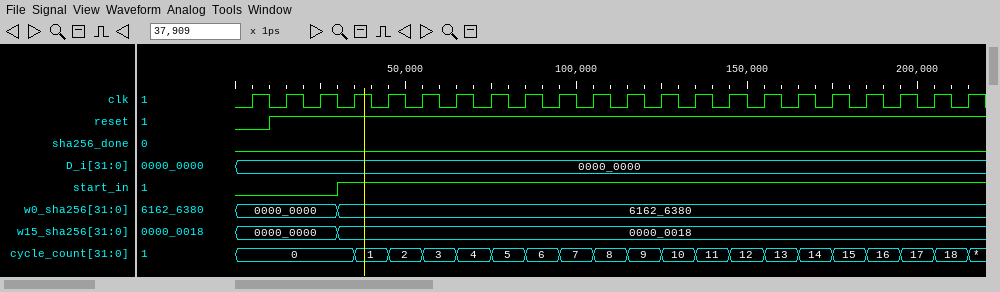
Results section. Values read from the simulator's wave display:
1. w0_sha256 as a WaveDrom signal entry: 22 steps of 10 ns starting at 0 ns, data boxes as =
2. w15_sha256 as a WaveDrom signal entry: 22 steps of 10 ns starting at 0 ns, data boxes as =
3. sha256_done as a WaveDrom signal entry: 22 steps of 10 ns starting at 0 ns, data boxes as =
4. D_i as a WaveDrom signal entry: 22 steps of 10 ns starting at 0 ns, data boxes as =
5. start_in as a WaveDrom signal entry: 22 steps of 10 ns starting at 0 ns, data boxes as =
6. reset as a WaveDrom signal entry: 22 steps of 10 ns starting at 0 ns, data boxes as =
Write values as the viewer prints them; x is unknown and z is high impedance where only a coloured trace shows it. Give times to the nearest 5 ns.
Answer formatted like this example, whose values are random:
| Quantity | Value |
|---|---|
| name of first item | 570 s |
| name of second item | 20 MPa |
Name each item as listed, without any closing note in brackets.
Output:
| Quantity | Value |
|---|---|
| w0_sha256 as a WaveDrom signal entry: 22 steps of 10 ns starting at 0 ns, data boxes as = | {name: 'w0_sha256', wave: '=..=..................', data: '0000_0000 6162_6380'} |
| w15_sha256 as a WaveDrom signal entry: 22 steps of 10 ns starting at 0 ns, data boxes as = | {name: 'w15_sha256', wave: '=..=..................', data: '0000_0000 0000_0018'} |
| sha256_done as a WaveDrom signal entry: 22 steps of 10 ns starting at 0 ns, data boxes as = | {name: 'sha256_done', wave: '0.....................'} |
| D_i as a WaveDrom signal entry: 22 steps of 10 ns starting at 0 ns, data boxes as = | {name: 'D_i', wave: '=.....................', data: '0000_0000'} |
| start_in as a WaveDrom signal entry: 22 steps of 10 ns starting at 0 ns, data boxes as = | {name: 'start_in', wave: '0..1..................'} |
| reset as a WaveDrom signal entry: 22 steps of 10 ns starting at 0 ns, data boxes as = | {name: 'reset', wave: '01....................'} |
